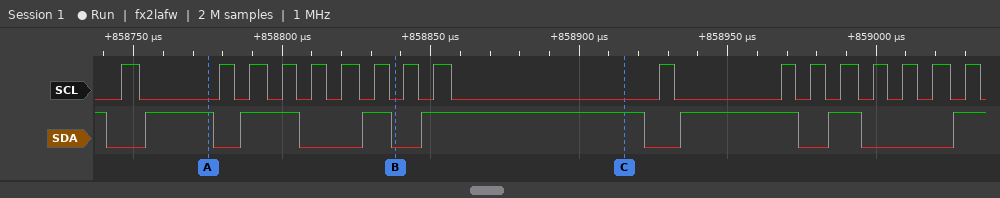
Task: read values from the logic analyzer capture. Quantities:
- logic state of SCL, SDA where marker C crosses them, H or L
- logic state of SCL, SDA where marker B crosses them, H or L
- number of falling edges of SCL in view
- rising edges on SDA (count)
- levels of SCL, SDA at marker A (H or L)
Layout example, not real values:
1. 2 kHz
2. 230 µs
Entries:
1. SCL=L, SDA=H
2. SCL=L, SDA=L
3. 17
4. 7
5. SCL=L, SDA=H
